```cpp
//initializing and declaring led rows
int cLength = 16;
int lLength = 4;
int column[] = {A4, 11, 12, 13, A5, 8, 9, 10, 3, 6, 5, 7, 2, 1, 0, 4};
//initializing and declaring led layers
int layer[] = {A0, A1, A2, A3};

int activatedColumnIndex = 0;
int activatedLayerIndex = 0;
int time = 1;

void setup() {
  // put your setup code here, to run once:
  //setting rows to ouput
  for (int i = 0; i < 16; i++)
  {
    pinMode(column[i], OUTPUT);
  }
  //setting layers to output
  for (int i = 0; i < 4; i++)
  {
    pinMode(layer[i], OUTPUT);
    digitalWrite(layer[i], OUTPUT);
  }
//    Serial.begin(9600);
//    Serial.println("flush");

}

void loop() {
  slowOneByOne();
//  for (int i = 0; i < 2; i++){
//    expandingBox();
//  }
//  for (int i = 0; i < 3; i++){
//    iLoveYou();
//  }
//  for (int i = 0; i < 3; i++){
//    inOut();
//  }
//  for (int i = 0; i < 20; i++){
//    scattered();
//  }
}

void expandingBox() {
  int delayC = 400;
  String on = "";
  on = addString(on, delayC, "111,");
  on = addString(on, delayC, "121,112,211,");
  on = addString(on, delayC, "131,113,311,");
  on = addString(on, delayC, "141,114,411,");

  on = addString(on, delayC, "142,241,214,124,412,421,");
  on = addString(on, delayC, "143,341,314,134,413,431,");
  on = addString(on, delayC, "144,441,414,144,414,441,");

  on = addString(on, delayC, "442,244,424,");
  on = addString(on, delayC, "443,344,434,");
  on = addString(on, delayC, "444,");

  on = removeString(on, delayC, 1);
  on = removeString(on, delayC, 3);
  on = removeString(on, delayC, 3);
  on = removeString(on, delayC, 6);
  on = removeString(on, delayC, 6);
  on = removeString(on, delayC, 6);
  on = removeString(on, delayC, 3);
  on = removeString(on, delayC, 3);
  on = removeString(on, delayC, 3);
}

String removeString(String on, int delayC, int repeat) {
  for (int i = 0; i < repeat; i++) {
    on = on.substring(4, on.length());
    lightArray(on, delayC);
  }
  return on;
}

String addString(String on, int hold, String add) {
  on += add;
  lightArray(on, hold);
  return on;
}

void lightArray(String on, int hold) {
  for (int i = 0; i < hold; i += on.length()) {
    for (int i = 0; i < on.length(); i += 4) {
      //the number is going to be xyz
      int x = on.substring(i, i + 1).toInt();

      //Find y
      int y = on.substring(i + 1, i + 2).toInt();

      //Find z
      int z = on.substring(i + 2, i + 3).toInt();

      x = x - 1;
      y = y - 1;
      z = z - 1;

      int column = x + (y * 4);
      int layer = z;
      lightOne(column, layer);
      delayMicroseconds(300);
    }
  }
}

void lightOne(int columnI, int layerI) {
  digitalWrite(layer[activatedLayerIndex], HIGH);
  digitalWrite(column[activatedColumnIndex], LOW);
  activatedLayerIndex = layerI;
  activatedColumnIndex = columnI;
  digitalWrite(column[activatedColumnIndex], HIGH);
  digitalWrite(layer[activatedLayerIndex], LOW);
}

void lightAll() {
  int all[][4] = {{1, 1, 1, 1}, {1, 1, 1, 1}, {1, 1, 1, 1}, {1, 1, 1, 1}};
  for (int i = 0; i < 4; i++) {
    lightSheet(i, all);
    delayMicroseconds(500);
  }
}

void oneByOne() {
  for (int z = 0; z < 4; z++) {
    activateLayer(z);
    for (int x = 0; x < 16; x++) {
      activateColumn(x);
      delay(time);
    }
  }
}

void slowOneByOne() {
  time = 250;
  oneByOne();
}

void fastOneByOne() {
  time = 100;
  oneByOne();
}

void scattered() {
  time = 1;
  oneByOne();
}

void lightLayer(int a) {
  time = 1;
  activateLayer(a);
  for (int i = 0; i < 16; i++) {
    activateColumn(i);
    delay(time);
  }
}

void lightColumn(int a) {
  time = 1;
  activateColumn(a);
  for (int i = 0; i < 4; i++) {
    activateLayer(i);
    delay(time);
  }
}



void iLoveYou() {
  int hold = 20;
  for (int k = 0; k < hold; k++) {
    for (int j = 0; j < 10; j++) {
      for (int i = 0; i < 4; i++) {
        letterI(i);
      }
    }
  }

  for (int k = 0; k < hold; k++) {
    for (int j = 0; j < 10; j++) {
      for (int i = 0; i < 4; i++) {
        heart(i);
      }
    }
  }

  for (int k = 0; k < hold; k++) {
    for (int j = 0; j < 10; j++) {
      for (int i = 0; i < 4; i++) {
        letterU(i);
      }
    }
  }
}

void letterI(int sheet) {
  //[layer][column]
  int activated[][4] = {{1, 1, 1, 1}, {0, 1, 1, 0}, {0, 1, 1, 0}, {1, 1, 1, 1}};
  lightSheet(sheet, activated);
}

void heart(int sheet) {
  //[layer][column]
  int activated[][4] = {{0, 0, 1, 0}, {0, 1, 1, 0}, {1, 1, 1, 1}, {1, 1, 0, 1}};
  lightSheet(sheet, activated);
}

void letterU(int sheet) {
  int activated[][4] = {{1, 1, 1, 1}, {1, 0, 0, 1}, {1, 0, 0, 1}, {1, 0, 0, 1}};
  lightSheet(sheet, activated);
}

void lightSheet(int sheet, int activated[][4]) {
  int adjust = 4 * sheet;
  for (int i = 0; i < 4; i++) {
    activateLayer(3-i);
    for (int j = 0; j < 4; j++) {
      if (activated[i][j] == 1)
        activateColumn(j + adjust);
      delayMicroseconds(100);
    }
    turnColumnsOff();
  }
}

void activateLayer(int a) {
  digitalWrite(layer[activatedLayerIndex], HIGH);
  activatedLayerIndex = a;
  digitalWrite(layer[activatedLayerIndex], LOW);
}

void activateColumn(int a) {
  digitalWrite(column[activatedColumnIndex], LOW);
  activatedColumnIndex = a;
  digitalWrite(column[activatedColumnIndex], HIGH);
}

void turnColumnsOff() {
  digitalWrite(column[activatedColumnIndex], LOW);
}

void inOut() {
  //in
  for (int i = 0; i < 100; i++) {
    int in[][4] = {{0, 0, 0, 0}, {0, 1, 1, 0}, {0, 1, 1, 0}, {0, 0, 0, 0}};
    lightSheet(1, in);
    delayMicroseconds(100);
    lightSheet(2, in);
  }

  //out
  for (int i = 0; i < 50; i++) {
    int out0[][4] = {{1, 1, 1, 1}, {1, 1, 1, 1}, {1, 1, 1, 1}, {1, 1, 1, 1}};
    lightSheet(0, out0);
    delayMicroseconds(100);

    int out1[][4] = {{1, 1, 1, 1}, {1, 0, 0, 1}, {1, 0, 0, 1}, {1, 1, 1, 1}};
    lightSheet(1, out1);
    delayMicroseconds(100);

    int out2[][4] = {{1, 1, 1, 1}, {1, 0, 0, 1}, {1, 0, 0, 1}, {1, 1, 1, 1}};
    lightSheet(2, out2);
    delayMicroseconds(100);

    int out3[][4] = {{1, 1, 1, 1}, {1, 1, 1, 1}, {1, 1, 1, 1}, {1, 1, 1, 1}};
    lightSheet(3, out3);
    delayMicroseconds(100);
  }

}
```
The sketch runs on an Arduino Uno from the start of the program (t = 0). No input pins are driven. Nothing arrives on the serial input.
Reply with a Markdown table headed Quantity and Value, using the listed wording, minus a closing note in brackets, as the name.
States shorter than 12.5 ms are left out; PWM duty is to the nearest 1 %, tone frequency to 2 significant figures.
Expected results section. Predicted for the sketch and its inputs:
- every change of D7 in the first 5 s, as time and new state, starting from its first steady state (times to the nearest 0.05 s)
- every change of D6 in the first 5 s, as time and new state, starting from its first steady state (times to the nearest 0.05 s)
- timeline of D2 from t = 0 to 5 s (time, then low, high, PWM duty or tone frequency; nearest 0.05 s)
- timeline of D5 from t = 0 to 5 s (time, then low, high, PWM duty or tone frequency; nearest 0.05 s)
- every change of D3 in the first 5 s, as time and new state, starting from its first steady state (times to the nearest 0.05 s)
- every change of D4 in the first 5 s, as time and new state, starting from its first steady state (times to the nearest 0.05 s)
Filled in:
| Quantity | Value |
|---|---|
| every change of D7 in the first 5 s, as time and new state, starting from its first steady state | 0 s low; 2.75 s high; 3 s low |
| every change of D6 in the first 5 s, as time and new state, starting from its first steady state | 0 s low; 2.25 s high; 2.5 s low |
| timeline of D2 from t = 0 to 5 s | 0 s low; 3 s high; 3.25 s low |
| timeline of D5 from t = 0 to 5 s | 0 s low; 2.5 s high; 2.75 s low |
| every change of D3 in the first 5 s, as time and new state, starting from its first steady state | 0 s low; 2 s high; 2.25 s low |
| every change of D4 in the first 5 s, as time and new state, starting from its first steady state | 0 s low; 3.75 s high; 4 s low |
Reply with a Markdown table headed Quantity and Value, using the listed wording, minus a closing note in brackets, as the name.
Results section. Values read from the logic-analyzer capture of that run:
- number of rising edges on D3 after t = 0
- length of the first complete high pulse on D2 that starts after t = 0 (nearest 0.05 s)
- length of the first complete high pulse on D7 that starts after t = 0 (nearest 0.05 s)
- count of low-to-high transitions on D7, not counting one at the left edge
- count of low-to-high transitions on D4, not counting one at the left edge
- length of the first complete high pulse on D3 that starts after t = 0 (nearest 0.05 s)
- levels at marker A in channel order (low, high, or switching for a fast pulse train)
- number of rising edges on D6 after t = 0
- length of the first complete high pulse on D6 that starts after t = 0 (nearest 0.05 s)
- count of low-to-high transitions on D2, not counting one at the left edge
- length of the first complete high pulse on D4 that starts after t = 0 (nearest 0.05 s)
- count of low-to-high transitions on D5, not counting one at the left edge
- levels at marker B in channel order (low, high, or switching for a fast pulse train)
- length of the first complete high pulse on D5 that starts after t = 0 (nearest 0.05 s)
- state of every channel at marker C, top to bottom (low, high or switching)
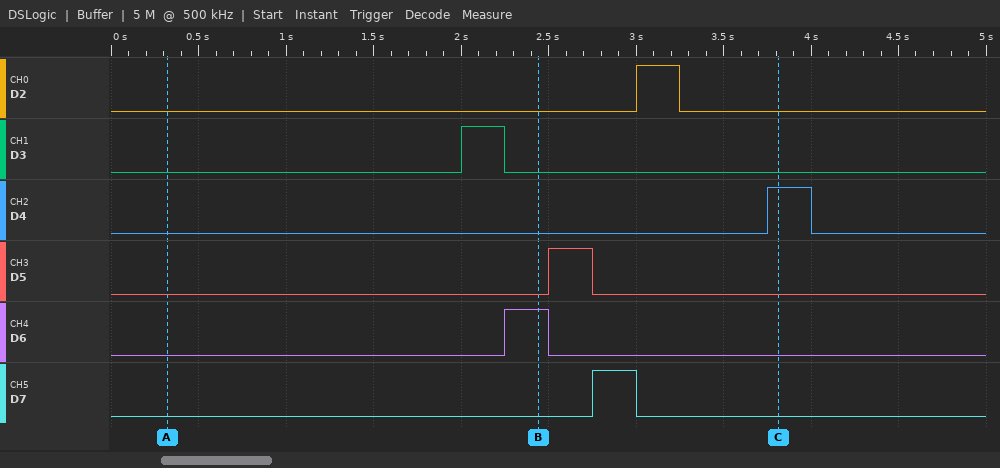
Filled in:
| Quantity | Value |
|---|---|
| number of rising edges on D3 after t = 0 | 1 |
| length of the first complete high pulse on D2 that starts after t = 0 | 0.25 s |
| length of the first complete high pulse on D7 that starts after t = 0 | 0.25 s |
| count of low-to-high transitions on D7, not counting one at the left edge | 1 |
| count of low-to-high transitions on D4, not counting one at the left edge | 1 |
| length of the first complete high pulse on D3 that starts after t = 0 | 0.25 s |
| levels at marker A in channel order | D2 low, D3 low, D4 low, D5 low, D6 low, D7 low |
| number of rising edges on D6 after t = 0 | 1 |
| length of the first complete high pulse on D6 that starts after t = 0 | 0.25 s |
| count of low-to-high transitions on D2, not counting one at the left edge | 1 |
| length of the first complete high pulse on D4 that starts after t = 0 | 0.25 s |
| count of low-to-high transitions on D5, not counting one at the left edge | 1 |
| levels at marker B in channel order | D2 low, D3 low, D4 low, D5 low, D6 high, D7 low |
| length of the first complete high pulse on D5 that starts after t = 0 | 0.25 s |
| state of every channel at marker C, top to bottom | D2 low, D3 low, D4 high, D5 low, D6 low, D7 low |
